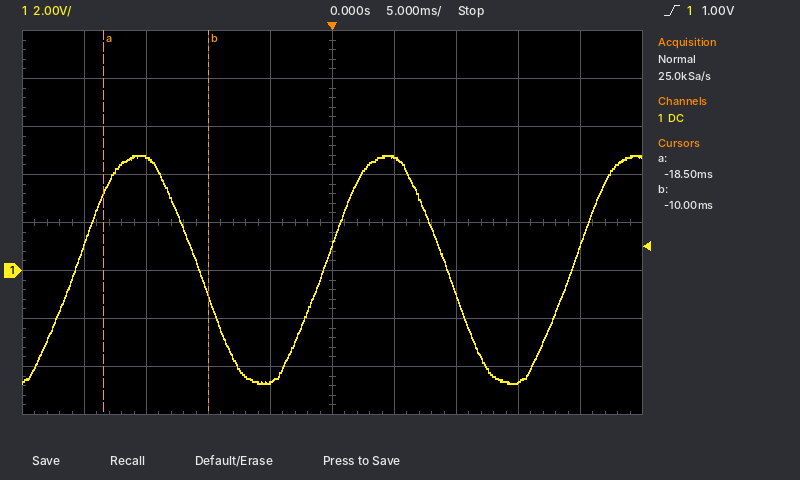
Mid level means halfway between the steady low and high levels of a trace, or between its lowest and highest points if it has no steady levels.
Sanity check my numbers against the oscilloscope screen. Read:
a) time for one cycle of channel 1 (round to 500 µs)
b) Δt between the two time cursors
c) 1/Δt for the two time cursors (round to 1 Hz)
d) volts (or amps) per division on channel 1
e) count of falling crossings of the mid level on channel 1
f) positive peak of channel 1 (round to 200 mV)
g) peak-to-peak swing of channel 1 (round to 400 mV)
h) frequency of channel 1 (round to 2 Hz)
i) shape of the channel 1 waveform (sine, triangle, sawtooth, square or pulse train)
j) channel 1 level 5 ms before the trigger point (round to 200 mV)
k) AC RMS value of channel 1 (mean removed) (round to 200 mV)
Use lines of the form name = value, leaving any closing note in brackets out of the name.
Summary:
time for one cycle of channel 1 = 20.0 ms
Δt between the two time cursors = 8.5 ms
1/Δt for the two time cursors = 118 Hz
volts (or amps) per division on channel 1 = 2 V
count of falling crossings of the mid level on channel 1 = 2
positive peak of channel 1 = 4.8 V
peak-to-peak swing of channel 1 = 9.6 V
frequency of channel 1 = 50 Hz
shape of the channel 1 waveform = sine
channel 1 level 5 ms before the trigger point = -4.6 V
AC RMS value of channel 1 (mean removed) = 3.4 V
